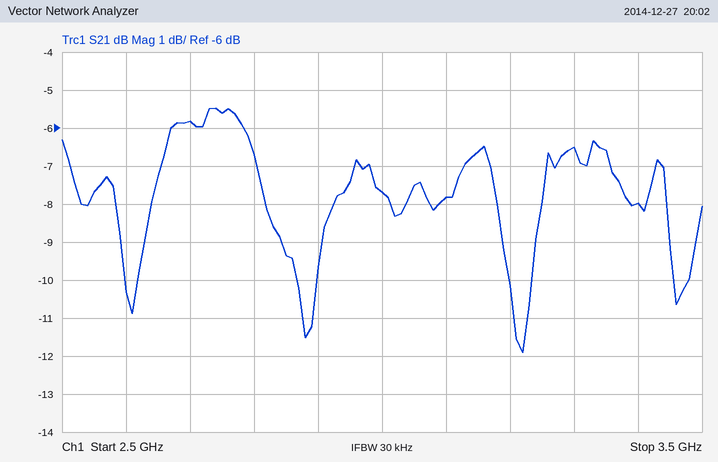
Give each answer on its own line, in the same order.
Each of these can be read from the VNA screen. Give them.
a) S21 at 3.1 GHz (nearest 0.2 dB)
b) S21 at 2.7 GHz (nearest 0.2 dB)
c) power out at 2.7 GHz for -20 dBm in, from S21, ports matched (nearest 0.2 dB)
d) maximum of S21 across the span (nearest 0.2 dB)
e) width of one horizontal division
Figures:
-7.8 dB
-5.8 dB
-25.8 dBm
-5.4 dB
100 MHz
